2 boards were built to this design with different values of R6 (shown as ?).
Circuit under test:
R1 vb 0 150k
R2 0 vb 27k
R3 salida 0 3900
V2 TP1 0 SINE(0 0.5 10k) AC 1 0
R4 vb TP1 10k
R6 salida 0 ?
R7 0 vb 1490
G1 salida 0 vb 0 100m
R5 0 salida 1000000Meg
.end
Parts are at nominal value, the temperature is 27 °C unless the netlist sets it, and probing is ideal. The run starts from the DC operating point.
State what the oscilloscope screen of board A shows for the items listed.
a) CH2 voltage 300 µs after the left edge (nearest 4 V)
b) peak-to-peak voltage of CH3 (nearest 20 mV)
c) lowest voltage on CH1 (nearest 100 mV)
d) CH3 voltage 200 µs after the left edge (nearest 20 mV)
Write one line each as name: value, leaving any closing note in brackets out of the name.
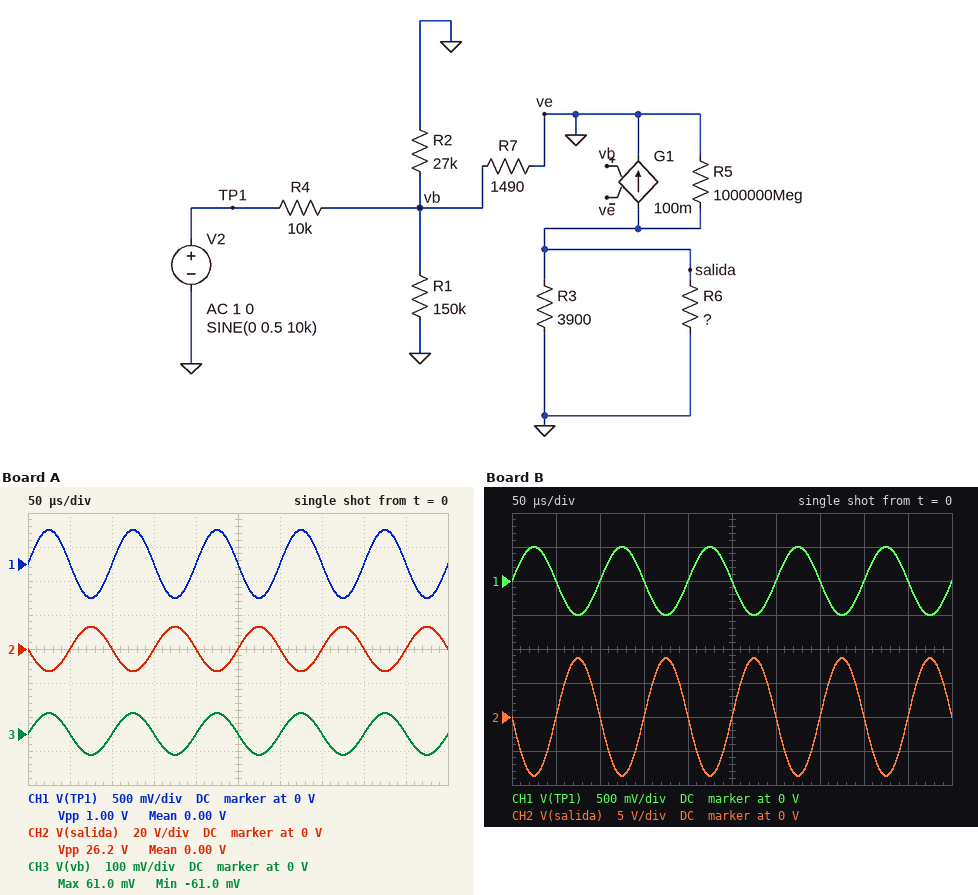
CH2 voltage 300 µs after the left edge: 0 V
peak-to-peak voltage of CH3: 120 mV
lowest voltage on CH1: -500 mV
CH3 voltage 200 µs after the left edge: 0 V
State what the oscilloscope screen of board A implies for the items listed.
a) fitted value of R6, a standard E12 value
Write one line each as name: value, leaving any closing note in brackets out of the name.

fitted value of R6, a standard E12 value: 4.7 kΩ
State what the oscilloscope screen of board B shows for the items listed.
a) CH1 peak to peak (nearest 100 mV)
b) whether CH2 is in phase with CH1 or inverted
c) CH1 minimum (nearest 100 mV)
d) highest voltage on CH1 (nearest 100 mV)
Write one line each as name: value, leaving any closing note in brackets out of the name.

CH1 peak to peak: 1.0 V
whether CH2 is in phase with CH1 or inverted: inverted
CH1 minimum: -500 mV
highest voltage on CH1: 500 mV
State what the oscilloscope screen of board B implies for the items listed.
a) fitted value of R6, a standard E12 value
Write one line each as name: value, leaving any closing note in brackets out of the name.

fitted value of R6, a standard E12 value: 2.2 kΩ
